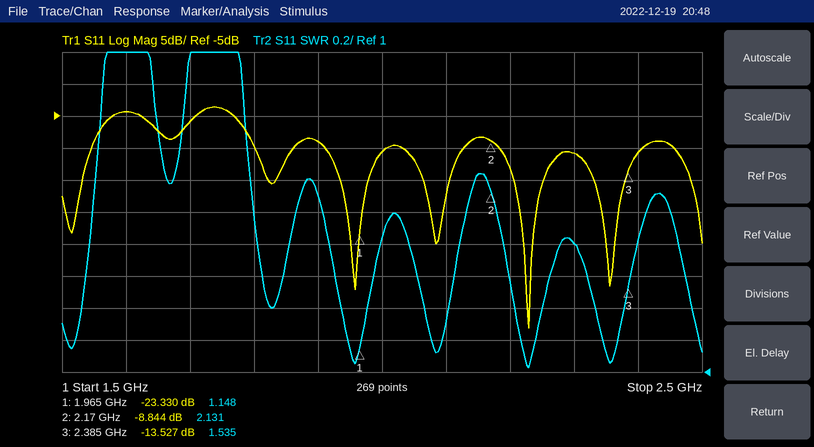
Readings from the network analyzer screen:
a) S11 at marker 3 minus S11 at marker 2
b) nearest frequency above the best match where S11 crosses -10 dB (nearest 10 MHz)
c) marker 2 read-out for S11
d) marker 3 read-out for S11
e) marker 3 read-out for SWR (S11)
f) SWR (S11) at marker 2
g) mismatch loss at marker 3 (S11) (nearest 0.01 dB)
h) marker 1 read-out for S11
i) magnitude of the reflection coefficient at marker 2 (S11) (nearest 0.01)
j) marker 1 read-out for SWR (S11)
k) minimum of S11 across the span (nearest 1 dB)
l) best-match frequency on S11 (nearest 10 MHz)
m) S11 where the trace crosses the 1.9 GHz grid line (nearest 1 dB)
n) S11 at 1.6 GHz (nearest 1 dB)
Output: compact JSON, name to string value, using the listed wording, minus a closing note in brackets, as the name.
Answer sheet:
{"S11 at marker 3 minus S11 at marker 2": "-4.683 dB", "nearest frequency above the best match where S11 crosses -10 dB": "2.41 GHz", "marker 2 read-out for S11": "-8.844 dB", "marker 3 read-out for S11": "-13.527 dB", "marker 3 read-out for SWR": "1.535", "SWR (S11) at marker 2": "2.131", "mismatch loss at marker 3 (S11)": "0.20 dB", "marker 1 read-out for S11": "-23.330 dB", "magnitude of the reflection coefficient at marker 2 (S11)": "0.36", "marker 1 read-out for SWR": "1.148", "minimum of S11 across the span": "-38 dB", "best-match frequency on S11": "2.23 GHz", "S11 where the trace crosses the 1.9 GHz grid line": "-9 dB", "S11 at 1.6 GHz": "-4 dB"}
